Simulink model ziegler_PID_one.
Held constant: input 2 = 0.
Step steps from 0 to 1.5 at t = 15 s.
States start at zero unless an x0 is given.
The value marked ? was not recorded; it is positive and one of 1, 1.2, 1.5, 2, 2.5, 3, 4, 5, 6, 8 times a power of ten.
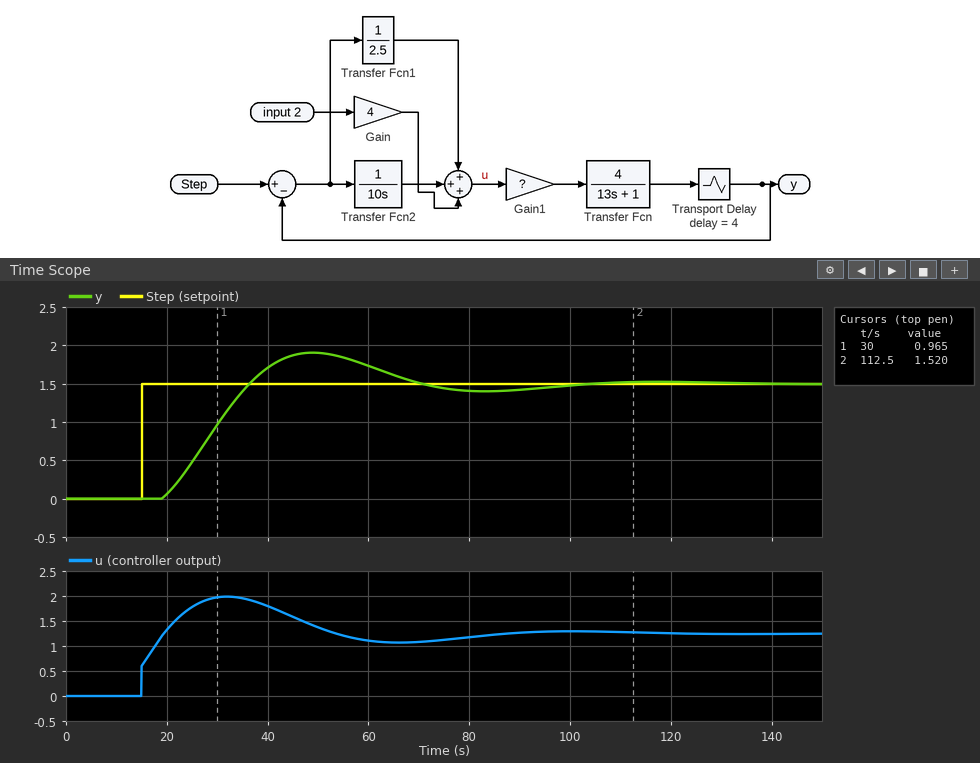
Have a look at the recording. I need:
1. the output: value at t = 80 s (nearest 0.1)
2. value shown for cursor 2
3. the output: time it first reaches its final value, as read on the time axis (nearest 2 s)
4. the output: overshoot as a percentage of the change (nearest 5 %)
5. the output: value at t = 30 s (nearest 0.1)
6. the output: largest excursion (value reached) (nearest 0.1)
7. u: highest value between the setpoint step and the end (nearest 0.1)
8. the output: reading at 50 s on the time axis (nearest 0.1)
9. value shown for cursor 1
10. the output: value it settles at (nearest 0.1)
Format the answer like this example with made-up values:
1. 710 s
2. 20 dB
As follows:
1. 1.4
2. 1.520
3. 36 s
4. 25 %
5. 1.0
6. 1.9
7. 2.0
8. 1.9
9. 0.965
10. 1.5
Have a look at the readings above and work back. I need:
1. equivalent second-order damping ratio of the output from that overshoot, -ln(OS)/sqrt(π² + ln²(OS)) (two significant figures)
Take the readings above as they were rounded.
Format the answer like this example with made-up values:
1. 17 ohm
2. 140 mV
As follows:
1. 0.40
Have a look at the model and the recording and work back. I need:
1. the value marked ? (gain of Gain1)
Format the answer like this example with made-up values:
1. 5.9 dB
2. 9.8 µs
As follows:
1. 0.3
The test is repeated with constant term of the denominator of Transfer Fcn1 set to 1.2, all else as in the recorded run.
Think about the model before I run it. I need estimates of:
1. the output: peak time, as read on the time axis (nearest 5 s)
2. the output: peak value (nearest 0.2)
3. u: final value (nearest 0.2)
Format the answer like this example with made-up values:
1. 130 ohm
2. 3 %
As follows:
1. 45 s
2. 1.6
3. 1.2
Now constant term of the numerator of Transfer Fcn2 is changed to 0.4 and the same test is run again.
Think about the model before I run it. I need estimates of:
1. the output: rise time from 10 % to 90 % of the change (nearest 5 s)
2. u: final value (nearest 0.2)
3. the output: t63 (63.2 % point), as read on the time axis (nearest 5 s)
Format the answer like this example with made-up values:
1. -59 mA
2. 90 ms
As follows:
1. 35 s
2. 1.2
3. 40 s
